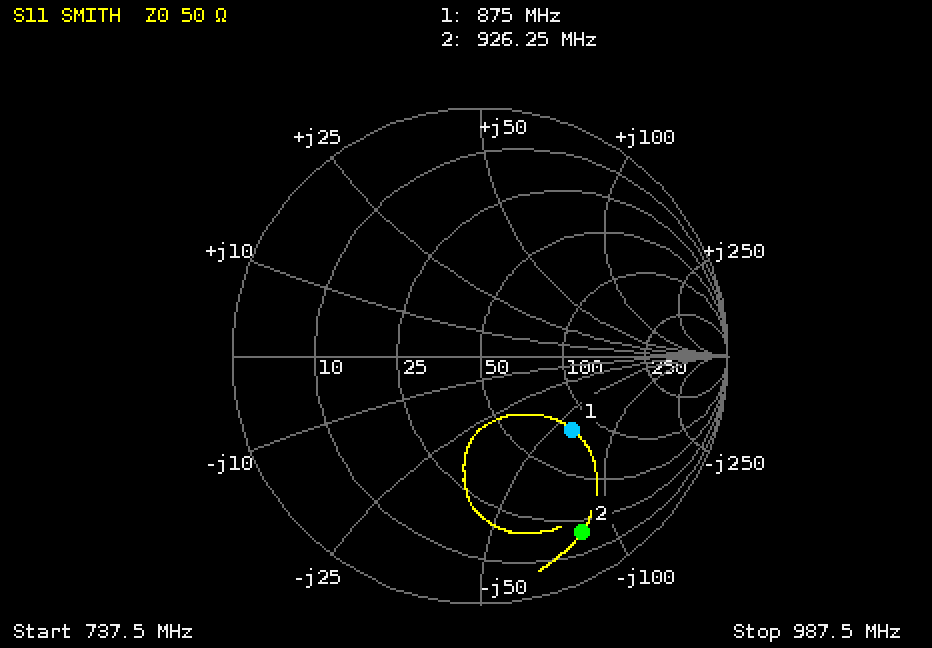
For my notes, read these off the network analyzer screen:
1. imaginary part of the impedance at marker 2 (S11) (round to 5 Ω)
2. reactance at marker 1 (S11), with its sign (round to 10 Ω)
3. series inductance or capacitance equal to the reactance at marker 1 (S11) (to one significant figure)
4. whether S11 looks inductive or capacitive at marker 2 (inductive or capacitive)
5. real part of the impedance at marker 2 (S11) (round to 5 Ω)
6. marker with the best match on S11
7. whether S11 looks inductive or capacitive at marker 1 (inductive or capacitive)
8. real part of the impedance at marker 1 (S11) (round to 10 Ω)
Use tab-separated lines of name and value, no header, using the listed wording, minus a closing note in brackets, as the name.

imaginary part of the impedance at marker 2 (S11)	-85 Ω
reactance at marker 1 (S11), with its sign	-60 Ω
series inductance or capacitance equal to the reactance at marker 1 (S11)	3 pF
whether S11 looks inductive or capacitive at marker 2	capacitive
real part of the impedance at marker 2 (S11)	20 Ω
marker with the best match on S11	marker 1
whether S11 looks inductive or capacitive at marker 1	capacitive
real part of the impedance at marker 1 (S11)	80 Ω
